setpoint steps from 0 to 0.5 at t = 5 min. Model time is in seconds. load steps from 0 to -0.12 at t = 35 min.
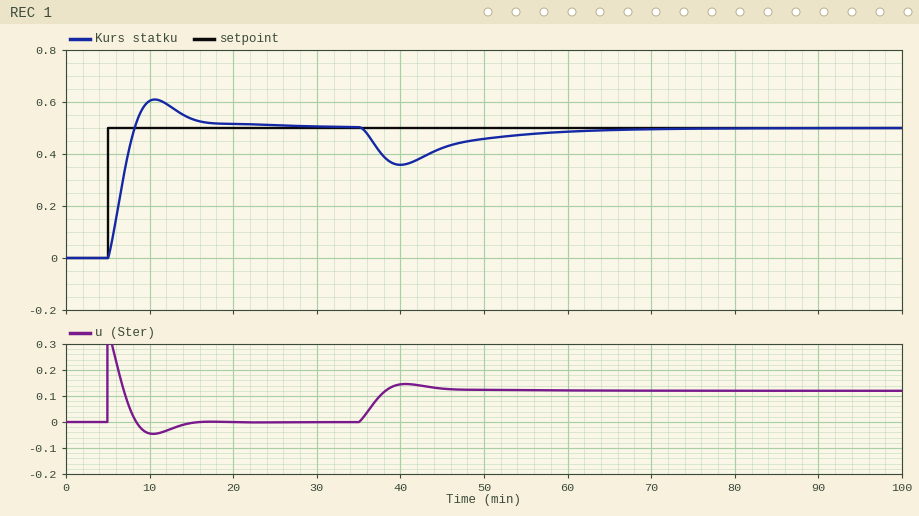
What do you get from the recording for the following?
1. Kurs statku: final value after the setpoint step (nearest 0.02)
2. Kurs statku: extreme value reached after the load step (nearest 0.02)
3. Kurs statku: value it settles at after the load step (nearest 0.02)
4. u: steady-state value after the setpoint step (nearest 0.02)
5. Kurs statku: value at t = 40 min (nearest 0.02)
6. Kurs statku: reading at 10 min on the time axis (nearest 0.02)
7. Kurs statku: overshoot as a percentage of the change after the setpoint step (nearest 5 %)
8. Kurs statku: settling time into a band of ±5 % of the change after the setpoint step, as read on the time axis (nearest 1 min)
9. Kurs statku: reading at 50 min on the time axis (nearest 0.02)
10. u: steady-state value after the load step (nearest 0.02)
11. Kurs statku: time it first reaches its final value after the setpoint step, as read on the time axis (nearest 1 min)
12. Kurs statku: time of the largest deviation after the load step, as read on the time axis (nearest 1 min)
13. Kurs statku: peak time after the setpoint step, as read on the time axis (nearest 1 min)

0.50
0.36
0.50
0.00
0.36
0.60
20 %
16 min
0.46
0.12
8 min
40 min
11 min
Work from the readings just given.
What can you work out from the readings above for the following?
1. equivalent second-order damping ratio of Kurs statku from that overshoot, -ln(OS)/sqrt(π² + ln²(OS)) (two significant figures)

0.46
